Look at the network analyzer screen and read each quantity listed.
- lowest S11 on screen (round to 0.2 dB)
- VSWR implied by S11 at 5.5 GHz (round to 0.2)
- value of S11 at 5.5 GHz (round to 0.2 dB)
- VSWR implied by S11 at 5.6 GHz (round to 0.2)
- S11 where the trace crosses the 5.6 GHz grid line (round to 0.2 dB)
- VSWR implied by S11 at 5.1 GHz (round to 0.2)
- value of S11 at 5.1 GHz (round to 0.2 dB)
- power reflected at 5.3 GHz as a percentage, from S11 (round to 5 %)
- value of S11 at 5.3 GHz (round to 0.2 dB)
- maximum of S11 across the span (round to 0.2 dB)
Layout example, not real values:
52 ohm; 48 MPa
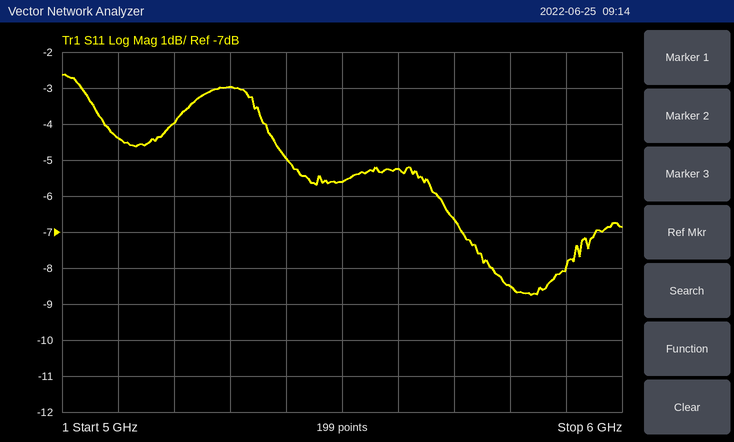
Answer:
-8.8 dB; 3.2; -5.6 dB; 3.4; -5.2 dB; 4.0; -4.4 dB; 50 %; -3.0 dB; -2.6 dB
